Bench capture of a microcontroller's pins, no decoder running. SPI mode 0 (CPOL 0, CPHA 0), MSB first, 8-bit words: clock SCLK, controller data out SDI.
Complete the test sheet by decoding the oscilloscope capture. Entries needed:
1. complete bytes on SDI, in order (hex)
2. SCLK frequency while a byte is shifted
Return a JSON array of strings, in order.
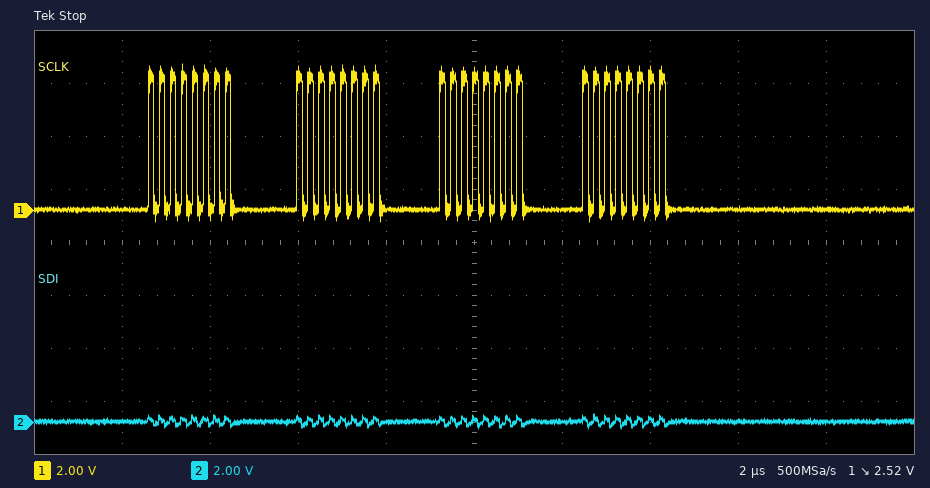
["00 00 00 00", "4 MHz"]
